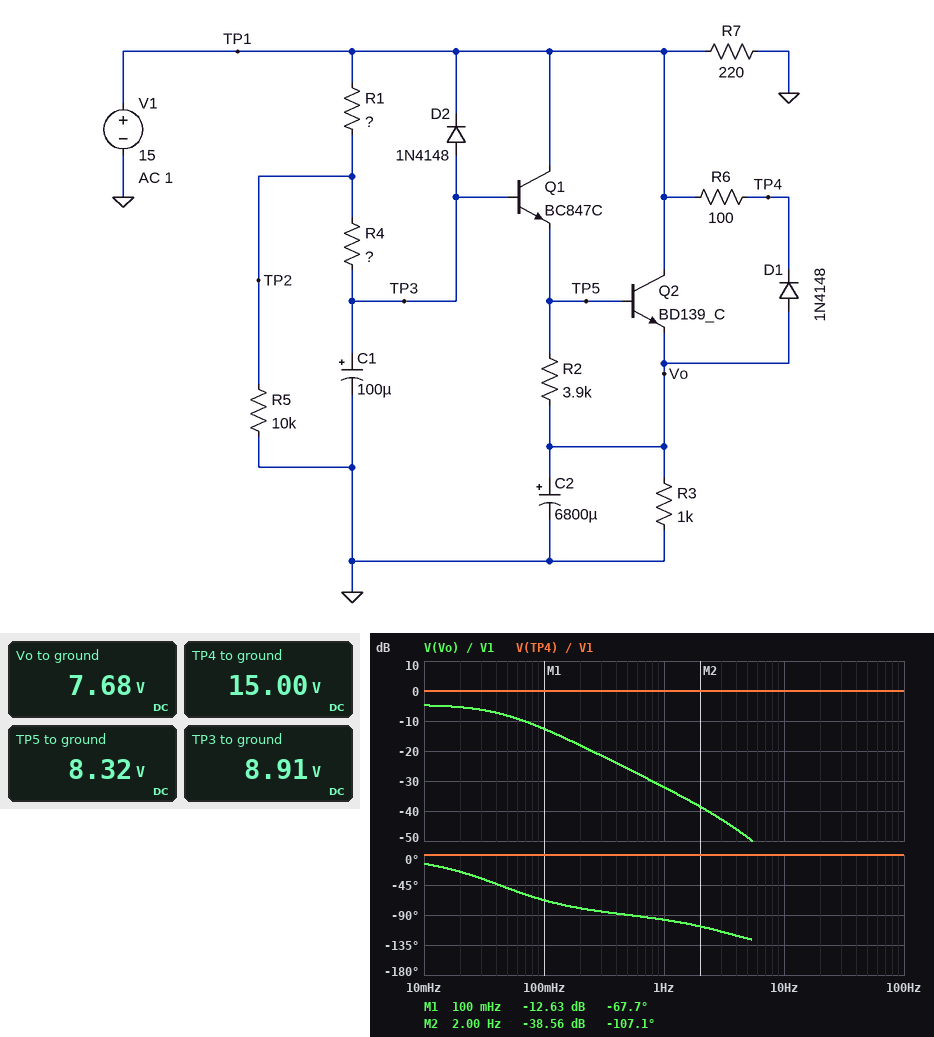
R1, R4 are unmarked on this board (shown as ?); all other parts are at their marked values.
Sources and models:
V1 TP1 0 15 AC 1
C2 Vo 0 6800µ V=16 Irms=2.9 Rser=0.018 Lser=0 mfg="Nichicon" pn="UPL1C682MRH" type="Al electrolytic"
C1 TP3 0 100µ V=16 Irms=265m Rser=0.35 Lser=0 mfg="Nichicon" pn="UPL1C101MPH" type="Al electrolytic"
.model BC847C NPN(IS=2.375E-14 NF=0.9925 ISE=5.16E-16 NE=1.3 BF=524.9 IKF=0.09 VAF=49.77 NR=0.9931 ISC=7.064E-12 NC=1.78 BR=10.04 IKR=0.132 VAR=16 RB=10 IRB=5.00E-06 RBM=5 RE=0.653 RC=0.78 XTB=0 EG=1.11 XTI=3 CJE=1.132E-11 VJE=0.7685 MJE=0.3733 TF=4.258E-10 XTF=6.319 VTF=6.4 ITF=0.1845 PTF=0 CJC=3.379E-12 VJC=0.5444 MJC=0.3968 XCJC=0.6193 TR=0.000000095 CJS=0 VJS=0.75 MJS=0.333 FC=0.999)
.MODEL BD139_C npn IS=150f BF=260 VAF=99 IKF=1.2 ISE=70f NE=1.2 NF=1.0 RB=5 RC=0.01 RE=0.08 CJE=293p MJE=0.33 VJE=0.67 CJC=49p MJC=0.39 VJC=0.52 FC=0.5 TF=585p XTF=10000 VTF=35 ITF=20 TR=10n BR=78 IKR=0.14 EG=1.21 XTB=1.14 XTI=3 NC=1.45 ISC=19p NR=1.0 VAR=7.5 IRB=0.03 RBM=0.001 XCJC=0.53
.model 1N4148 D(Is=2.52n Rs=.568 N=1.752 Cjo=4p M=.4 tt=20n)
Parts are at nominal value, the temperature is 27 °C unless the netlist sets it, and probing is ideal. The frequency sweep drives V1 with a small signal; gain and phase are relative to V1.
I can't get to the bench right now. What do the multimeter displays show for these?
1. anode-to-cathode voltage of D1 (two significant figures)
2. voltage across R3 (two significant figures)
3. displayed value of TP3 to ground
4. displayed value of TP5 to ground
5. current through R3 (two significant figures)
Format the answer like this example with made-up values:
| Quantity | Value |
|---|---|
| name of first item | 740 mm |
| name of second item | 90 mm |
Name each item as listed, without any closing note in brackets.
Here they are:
| Quantity | Value |
|---|---|
| anode-to-cathode voltage of D1 | -7.3 V |
| voltage across R3 | 7.7 V |
| displayed value of TP3 to ground | 8.91 V |
| displayed value of TP5 to ground | 8.32 V |
| current through R3 | 7.7 mA |
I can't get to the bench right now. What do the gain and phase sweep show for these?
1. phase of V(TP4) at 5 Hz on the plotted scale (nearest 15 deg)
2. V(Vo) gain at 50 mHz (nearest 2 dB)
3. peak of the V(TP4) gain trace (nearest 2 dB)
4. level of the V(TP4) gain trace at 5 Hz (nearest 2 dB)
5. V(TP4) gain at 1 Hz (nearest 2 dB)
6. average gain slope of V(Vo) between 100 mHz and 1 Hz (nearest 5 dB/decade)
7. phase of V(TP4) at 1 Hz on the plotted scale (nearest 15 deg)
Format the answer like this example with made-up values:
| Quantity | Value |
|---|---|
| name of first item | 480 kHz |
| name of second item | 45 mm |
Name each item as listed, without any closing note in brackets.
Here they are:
| Quantity | Value |
|---|---|
| phase of V(TP4) at 5 Hz on the plotted scale | 0 deg |
| V(Vo) gain at 50 mHz | -8 dB |
| peak of the V(TP4) gain trace | 0 dB |
| level of the V(TP4) gain trace at 5 Hz | 0 dB |
| V(TP4) gain at 1 Hz | 0 dB |
| average gain slope of V(Vo) between 100 mHz and 1 Hz | -20 dB/decade |
| phase of V(TP4) at 1 Hz on the plotted scale | 0 deg |
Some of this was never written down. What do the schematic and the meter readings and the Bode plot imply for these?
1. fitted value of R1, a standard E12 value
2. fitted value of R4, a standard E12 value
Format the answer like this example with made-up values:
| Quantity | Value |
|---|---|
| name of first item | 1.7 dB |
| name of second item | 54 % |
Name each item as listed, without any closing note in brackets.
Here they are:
| Quantity | Value |
|---|---|
| fitted value of R1, a standard E12 value | 6.8 kΩ |
| fitted value of R4, a standard E12 value | 33 kΩ |
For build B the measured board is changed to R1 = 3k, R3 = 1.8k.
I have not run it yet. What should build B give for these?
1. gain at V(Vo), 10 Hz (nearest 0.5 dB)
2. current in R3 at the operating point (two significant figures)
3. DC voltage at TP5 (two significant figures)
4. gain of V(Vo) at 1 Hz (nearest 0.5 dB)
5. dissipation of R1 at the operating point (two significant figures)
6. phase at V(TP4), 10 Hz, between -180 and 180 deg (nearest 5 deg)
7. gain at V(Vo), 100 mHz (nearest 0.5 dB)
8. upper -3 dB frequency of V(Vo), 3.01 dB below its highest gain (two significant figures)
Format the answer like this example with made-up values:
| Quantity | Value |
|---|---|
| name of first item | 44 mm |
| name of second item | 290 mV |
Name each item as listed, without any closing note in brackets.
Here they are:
| Quantity | Value |
|---|---|
| gain at V(Vo), 10 Hz | -58.0 dB |
| current in R3 at the operating point | 5.7 mA |
| DC voltage at TP5 | 11 V |
| gain of V(Vo) at 1 Hz | -29.5 dB |
| dissipation of R1 at the operating point | 4.0 mW |
| phase at V(TP4), 10 Hz, between -180 and 180 deg | 0 deg |
| gain at V(Vo), 100 mHz | -10.0 dB |
| upper -3 dB frequency of V(Vo), 3.01 dB below its highest gain | 45 mHz |
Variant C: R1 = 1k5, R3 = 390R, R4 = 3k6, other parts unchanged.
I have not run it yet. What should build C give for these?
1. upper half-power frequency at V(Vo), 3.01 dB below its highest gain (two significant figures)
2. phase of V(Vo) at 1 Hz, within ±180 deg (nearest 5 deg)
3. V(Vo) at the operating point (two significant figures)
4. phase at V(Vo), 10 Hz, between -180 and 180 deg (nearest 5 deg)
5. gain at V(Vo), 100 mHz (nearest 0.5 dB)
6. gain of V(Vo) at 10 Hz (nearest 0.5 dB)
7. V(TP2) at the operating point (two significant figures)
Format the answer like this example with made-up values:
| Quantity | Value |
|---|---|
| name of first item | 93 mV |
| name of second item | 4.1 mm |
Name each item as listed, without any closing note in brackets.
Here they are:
| Quantity | Value |
|---|---|
| upper half-power frequency at V(Vo), 3.01 dB below its highest gain | 320 mHz |
| phase of V(Vo) at 1 Hz, within ±180 deg | -75 deg |
| V(Vo) at the operating point | 12 V |
| phase at V(Vo), 10 Hz, between -180 and 180 deg | -120 deg |
| gain at V(Vo), 100 mHz | -1.5 dB |
| gain of V(Vo) at 10 Hz | -32.5 dB |
| V(TP2) at the operating point | 13 V |
